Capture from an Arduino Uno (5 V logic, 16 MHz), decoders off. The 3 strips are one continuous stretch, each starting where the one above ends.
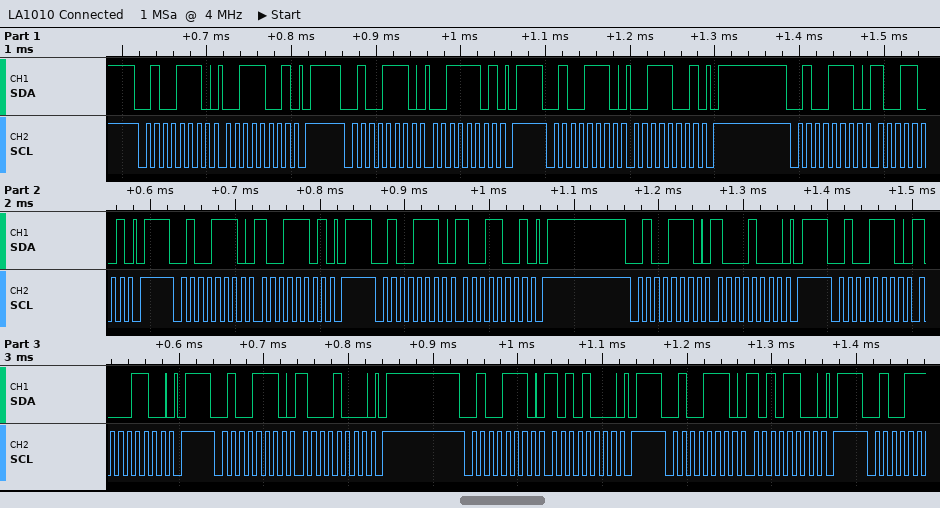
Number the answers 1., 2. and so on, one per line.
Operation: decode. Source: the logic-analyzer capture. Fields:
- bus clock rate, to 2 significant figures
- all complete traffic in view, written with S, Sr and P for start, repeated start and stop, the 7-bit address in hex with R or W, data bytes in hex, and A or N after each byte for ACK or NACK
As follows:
1. 100 kHz
2. S 27W A 39 A P S 27W A 3D A P S 27W A 39 A P S 27W A 99 A P S 27W A 9D A P S 27W A 99 A P S 27W A 88 A P S 27W A 8C A P S 27W A 88 A P S 27W A A8 A P S 27W A AC A P
